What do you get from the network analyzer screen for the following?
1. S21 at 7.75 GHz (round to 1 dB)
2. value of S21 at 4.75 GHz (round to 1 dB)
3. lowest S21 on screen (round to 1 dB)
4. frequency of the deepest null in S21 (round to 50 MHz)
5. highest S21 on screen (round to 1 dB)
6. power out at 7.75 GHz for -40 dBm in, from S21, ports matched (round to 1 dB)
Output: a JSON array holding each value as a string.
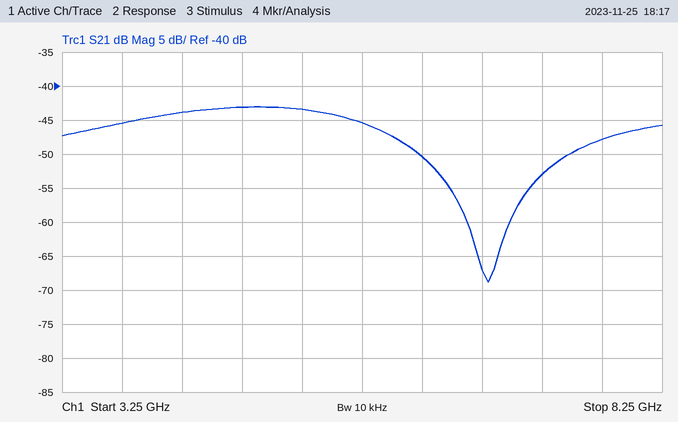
["-48 dB", "-43 dB", "-69 dB", "6.80 GHz", "-43 dB", "-88 dBm"]
